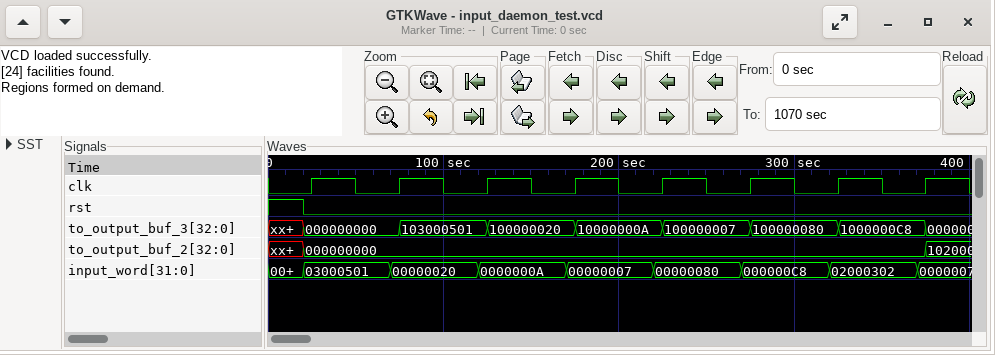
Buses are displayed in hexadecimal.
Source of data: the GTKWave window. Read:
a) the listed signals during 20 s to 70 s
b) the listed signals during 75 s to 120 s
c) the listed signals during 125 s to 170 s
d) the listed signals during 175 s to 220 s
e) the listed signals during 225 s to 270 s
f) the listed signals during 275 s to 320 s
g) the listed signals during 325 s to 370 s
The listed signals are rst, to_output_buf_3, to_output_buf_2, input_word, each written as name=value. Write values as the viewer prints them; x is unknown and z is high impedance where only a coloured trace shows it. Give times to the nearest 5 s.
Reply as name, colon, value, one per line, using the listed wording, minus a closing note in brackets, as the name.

the listed signals during 20 s to 70 s: rst=0, to_output_buf_3=000000000, to_output_buf_2=000000000, input_word=03000501
the listed signals during 75 s to 120 s: rst=0, to_output_buf_3=103000501, to_output_buf_2=000000000, input_word=00000020
the listed signals during 125 s to 170 s: rst=0, to_output_buf_3=100000020, to_output_buf_2=000000000, input_word=0000000A
the listed signals during 175 s to 220 s: rst=0, to_output_buf_3=10000000A, to_output_buf_2=000000000, input_word=00000007
the listed signals during 225 s to 270 s: rst=0, to_output_buf_3=100000007, to_output_buf_2=000000000, input_word=00000080
the listed signals during 275 s to 320 s: rst=0, to_output_buf_3=100000080, to_output_buf_2=000000000, input_word=000000C8
the listed signals during 325 s to 370 s: rst=0, to_output_buf_3=1000000C8, to_output_buf_2=000000000, input_word=02000302
